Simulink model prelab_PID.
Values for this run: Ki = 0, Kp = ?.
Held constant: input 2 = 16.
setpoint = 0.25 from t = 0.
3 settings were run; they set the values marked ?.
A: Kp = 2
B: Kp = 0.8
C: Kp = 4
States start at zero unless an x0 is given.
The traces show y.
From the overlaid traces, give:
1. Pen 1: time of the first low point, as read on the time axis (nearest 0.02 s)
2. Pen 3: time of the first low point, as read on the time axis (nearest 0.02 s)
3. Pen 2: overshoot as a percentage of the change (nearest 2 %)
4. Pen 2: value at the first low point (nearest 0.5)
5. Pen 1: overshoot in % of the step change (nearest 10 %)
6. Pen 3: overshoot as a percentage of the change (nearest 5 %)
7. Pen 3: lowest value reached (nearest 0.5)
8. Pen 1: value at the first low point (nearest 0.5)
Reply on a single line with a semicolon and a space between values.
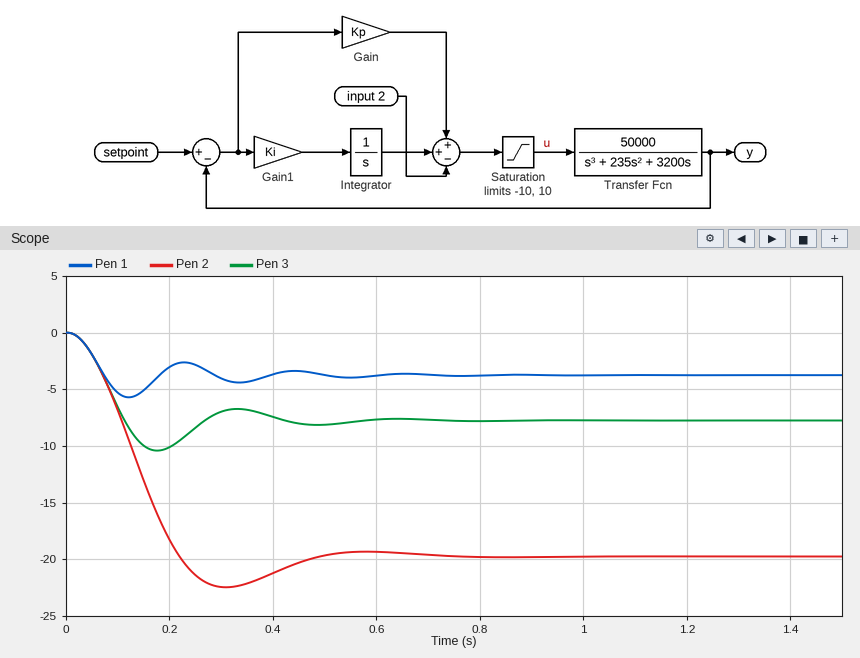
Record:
0.12 s; 0.18 s; 14 %; -22.5; 50 %; 35 %; -10.5; -5.5
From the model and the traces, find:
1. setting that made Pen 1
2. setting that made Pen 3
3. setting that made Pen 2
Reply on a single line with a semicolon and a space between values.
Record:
C; A; B
